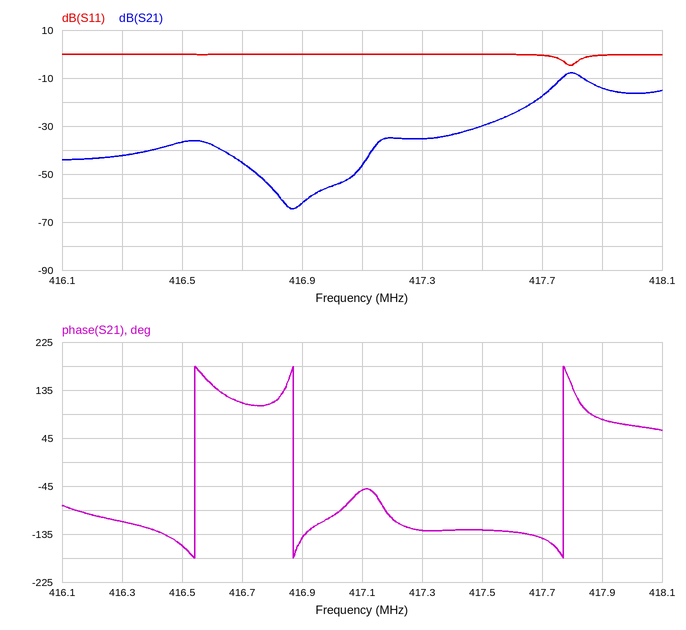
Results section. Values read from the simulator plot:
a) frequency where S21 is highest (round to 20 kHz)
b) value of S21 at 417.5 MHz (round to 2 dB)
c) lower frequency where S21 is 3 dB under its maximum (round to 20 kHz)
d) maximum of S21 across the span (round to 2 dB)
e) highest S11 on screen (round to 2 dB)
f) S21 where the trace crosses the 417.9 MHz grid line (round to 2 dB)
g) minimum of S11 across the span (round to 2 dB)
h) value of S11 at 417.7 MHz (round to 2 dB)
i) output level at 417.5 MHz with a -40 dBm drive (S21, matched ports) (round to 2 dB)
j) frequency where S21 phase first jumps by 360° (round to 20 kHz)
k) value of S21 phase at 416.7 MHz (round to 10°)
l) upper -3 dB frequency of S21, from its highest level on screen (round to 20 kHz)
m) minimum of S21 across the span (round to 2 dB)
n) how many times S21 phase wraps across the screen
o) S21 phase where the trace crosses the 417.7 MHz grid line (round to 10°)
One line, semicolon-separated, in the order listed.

417.80 MHz; -30 dB; 417.76 MHz; -8 dB; 0 dB; -14 dB; -4 dB; 0 dB; -70 dBm; 416.54 MHz; 110°; 417.84 MHz; -64 dB; 3; -140°
